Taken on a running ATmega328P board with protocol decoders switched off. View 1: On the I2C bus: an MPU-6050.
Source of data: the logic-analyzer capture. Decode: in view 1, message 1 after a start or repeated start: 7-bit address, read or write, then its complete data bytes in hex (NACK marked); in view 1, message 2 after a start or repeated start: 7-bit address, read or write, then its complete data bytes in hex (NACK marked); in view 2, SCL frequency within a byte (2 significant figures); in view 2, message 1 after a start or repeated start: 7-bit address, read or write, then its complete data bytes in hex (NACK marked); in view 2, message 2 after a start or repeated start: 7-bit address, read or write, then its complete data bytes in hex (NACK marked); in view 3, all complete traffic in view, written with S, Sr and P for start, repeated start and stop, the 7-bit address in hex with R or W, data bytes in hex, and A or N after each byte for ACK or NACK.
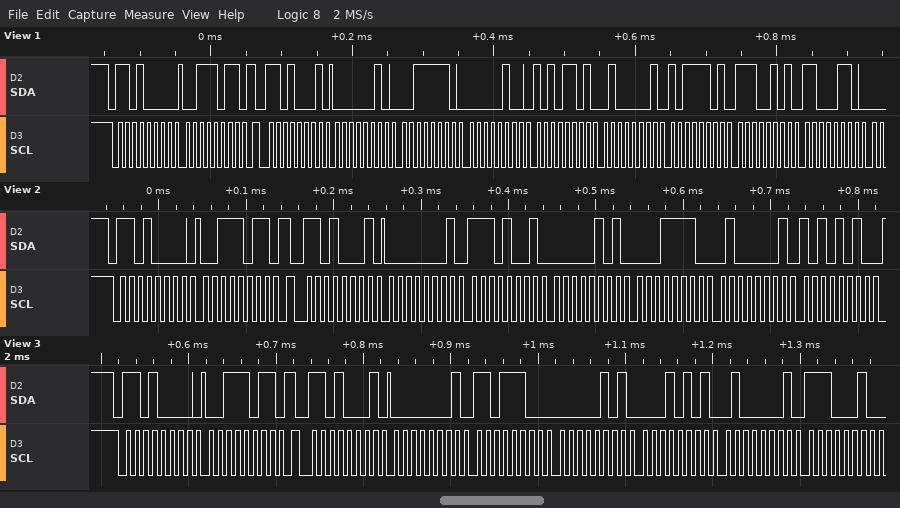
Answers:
0x68 write: 3B
0x68 read: 02 3E 04 AD 41 BD E5 C6
100 kHz
0x68 write: 3B
0x68 read: 01 E9 05 1E 41 AA
S 68W A 3B A Sr 68R A 01 A DC A 05 A 15 A 41 A E2 A
